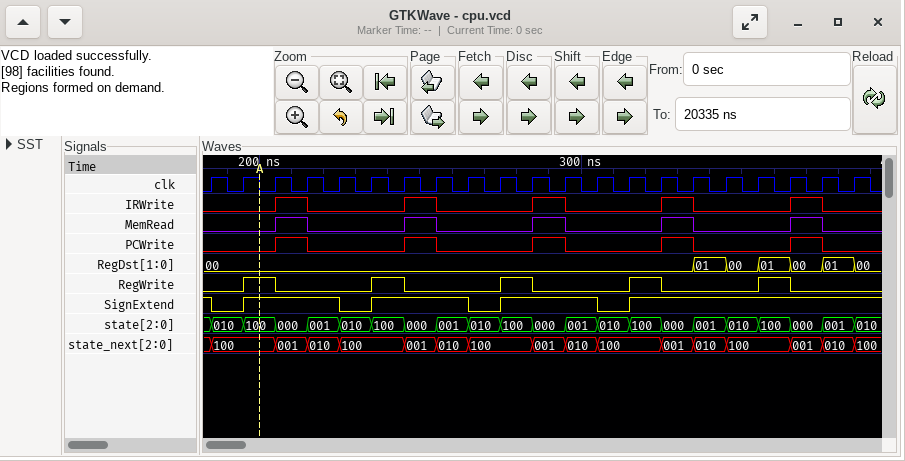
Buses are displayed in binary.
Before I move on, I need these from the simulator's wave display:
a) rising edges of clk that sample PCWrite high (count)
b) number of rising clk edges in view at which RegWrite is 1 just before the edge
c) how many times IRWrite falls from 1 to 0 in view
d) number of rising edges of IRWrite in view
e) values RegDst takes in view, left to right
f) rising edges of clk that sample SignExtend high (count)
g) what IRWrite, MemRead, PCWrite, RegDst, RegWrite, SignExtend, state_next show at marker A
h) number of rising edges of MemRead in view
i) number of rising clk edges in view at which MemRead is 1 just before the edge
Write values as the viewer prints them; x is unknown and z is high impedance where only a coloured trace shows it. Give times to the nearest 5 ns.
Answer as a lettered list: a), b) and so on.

a) 5
b) 5
c) 5
d) 5
e) 00, 01, 00, 01, 00, 01, 00
f) 17
g) IRWrite=0, MemRead=0, PCWrite=0, RegDst=00, RegWrite=1, SignExtend=1, state_next=100
h) 5
i) 5
